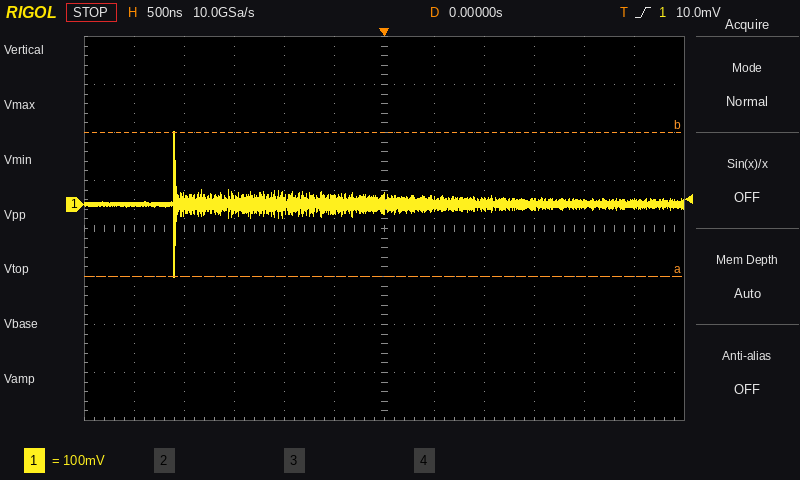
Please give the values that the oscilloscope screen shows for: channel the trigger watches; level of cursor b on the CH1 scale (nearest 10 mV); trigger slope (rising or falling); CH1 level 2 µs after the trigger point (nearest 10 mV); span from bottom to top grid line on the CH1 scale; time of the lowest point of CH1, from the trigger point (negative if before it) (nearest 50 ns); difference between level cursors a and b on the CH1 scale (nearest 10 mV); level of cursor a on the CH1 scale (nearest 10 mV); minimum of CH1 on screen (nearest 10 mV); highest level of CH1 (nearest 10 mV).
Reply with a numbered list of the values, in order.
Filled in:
1. CH1
2. 150 mV
3. rising
4. 0 mV
5. 800 mV
6. -2.10 µs
7. 300 mV
8. -150 mV
9. -150 mV
10. 150 mV
